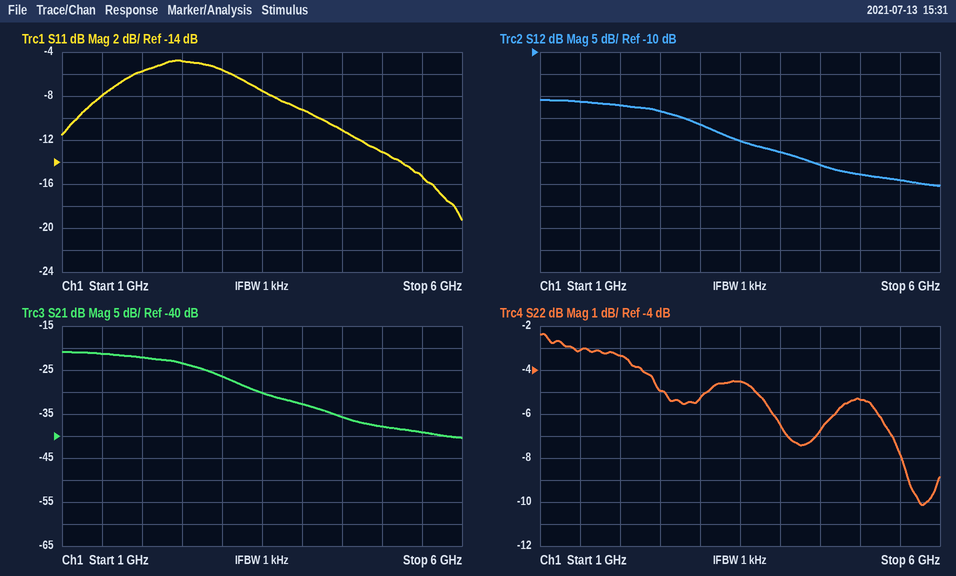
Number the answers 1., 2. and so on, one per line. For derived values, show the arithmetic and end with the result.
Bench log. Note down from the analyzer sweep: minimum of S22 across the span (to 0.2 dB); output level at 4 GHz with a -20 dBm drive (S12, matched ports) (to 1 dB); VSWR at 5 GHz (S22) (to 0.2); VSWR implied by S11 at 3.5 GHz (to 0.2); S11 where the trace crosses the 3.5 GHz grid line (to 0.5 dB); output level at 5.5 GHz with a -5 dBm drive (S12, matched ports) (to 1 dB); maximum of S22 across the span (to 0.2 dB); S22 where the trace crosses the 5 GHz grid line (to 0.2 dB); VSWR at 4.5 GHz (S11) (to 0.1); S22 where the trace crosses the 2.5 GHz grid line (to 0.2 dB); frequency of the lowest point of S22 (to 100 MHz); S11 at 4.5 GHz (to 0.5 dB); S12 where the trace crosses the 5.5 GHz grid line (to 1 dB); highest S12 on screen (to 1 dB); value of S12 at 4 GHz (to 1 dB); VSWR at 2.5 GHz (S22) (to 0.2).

1. -10.2 dB
2. -20 dBm + (-33 dB) = -53 dBm
3. |Γ| = 10^(-5.4/20) = 0.5370; VSWR = (1 + 0.5370)/(1 − 0.5370) ≈ 3.32, so 3.4 to the nearest 0.2
4. |Γ| = 10^(-7.5/20) = 0.4217; VSWR = (1 + 0.4217)/(1 − 0.4217) ≈ 2.46, so 2.4 to the nearest 0.2
5. -7.5 dB
6. -5 dBm + (-39 dB) = -44 dBm
7. -2.4 dB
8. -5.4 dB
9. |Γ| = 10^(-11/20) = 0.2818; VSWR = (1 + 0.2818)/(1 − 0.2818) ≈ 1.8
10. -5.0 dB
11. 5.8 GHz
12. -11.0 dB
13. -39 dB
14. -21 dB
15. -33 dB
16. |Γ| = 10^(-5/20) = 0.5623; VSWR = (1 + 0.5623)/(1 − 0.5623) ≈ 3.6
